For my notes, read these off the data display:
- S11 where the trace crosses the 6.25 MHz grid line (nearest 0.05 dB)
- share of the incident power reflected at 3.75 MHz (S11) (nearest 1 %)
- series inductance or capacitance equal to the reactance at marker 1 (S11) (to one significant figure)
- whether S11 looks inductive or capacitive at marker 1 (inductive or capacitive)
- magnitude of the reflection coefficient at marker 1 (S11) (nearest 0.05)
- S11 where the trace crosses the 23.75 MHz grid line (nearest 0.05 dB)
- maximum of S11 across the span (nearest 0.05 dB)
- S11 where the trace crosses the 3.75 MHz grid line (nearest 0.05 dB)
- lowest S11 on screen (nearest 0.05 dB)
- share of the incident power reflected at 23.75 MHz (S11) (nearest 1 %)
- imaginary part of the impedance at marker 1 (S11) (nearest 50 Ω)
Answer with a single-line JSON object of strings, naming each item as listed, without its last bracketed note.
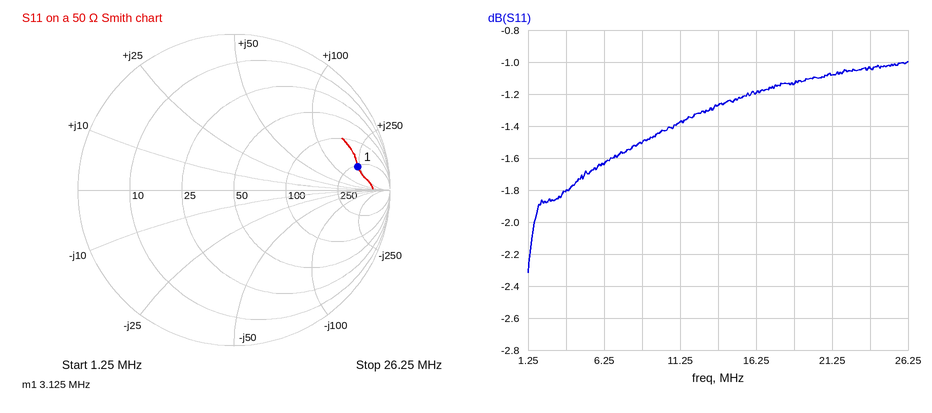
{"S11 where the trace crosses the 6.25 MHz grid line": "-1.65 dB", "share of the incident power reflected at 3.75 MHz (S11)": "66 %", "series inductance or capacitance equal to the reactance at marker 1 (S11)": "10 µH", "whether S11 looks inductive or capacitive at marker 1": "inductive", "magnitude of the reflection coefficient at marker 1 (S11)": "0.80", "S11 where the trace crosses the 23.75 MHz grid line": "-1.05 dB", "maximum of S11 across the span": "-1.00 dB", "S11 where the trace crosses the 3.75 MHz grid line": "-1.80 dB", "lowest S11 on screen": "-2.30 dB", "share of the incident power reflected at 23.75 MHz (S11)": "79 %", "imaginary part of the impedance at marker 1 (S11)": "+250 Ω"}
